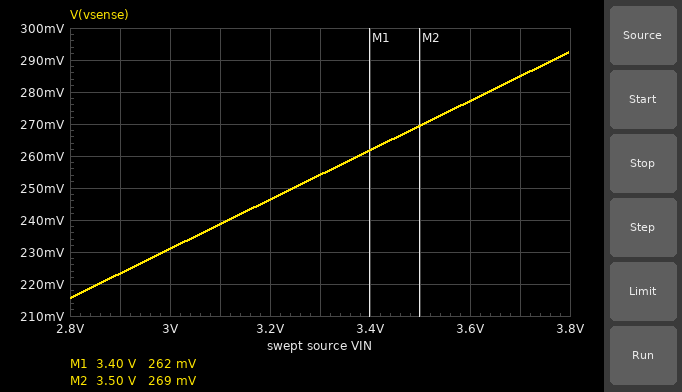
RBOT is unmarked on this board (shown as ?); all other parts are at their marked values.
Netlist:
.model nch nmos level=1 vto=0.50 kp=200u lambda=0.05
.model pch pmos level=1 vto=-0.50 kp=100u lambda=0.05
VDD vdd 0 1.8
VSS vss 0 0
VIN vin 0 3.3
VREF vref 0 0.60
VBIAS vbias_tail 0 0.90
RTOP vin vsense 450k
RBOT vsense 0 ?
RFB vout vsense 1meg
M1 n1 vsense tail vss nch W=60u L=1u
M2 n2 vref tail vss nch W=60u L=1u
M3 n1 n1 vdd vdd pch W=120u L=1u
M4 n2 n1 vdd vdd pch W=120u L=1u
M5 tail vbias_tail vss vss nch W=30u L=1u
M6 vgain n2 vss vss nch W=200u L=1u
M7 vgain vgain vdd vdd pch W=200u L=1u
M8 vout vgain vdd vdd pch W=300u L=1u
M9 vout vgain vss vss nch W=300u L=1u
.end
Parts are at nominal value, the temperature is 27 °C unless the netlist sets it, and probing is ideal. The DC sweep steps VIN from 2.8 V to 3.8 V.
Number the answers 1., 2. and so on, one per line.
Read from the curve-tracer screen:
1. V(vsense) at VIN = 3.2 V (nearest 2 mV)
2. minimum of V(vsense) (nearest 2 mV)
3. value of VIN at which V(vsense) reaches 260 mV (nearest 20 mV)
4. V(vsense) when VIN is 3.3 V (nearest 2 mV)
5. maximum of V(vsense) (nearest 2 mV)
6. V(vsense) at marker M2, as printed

1. 246 mV
2. 216 mV
3. 3.38 V
4. 254 mV
5. 292 mV
6. 269 mV
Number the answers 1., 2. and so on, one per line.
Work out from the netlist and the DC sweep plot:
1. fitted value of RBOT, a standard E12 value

1. 39 kΩ
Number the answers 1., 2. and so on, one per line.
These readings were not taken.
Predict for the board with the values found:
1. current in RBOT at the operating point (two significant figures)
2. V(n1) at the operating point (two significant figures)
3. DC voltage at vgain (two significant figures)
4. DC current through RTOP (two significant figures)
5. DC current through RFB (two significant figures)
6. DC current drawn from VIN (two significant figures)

1. 6.5 µA
2. 1.3 V
3. 1.3 V
4. 6.8 µA
5. 250 nA
6. 6.8 µA
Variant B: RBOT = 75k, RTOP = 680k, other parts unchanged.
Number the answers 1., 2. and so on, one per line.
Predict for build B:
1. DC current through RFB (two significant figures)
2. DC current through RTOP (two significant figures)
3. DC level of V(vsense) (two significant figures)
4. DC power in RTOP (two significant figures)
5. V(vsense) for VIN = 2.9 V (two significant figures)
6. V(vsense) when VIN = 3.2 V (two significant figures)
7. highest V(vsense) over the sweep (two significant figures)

1. 310 nA
2. 4.4 µA
3. 310 mV
4. 13 µW
5. 270 mV
6. 300 mV
7. 350 mV
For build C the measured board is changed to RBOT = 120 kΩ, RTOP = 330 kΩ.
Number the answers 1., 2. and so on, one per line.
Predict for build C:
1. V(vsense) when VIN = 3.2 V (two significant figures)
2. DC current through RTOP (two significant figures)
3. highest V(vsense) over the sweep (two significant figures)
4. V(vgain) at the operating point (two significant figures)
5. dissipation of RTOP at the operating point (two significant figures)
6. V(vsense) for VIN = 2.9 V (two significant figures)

1. 930 mV
2. 7.1 µA
3. 1.1 V
4. 250 mV
5. 17 µW
6. 860 mV
